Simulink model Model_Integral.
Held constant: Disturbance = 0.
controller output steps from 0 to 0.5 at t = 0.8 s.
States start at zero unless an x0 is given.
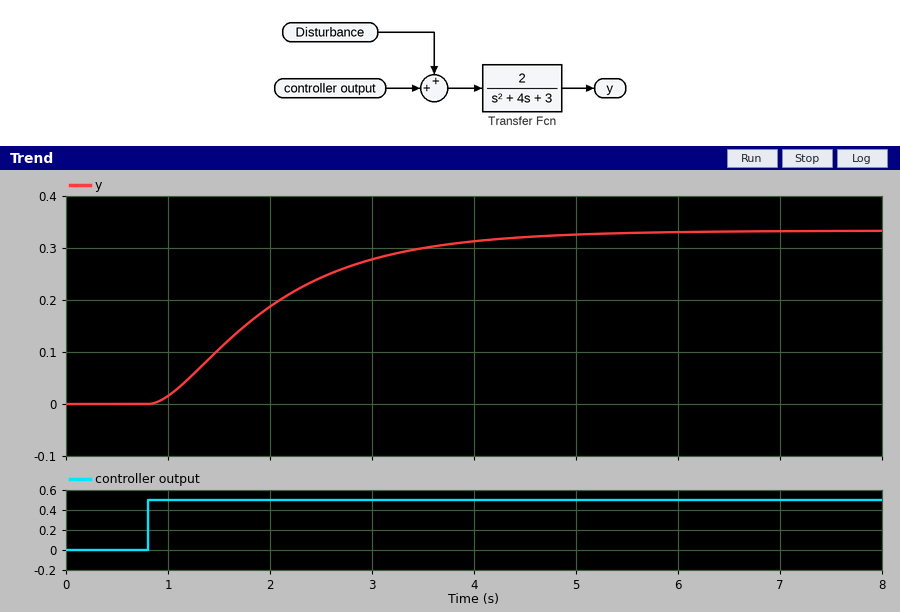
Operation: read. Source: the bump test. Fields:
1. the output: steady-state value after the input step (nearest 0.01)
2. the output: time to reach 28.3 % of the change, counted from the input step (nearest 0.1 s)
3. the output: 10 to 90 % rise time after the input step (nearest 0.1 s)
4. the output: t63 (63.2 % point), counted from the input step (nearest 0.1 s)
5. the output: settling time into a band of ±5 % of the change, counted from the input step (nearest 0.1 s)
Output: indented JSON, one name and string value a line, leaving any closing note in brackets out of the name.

{
  "the output: steady-state value after the input step": "0.33",
  "the output: time to reach 28.3 % of the change, counted from the input step": "0.6 s",
  "the output: 10 to 90 % rise time after the input step": "2.4 s",
  "the output: t63 (63.2 % point), counted from the input step": "1.4 s",
  "the output: settling time into a band of ±5 % of the change, counted from the input step": "3.4 s"
}
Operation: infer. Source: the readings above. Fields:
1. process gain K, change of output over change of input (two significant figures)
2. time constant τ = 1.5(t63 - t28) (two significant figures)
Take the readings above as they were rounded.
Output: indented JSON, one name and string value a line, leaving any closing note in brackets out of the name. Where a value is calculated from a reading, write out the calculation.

{
  "process gain K, change of output over change of input": "(0.33 - 0) / 0.5 = 0.66",
  "time constant τ = 1.5(t63 - t28)": "1.5 × (1.4 - 0.6) = 1.2 s"
}
